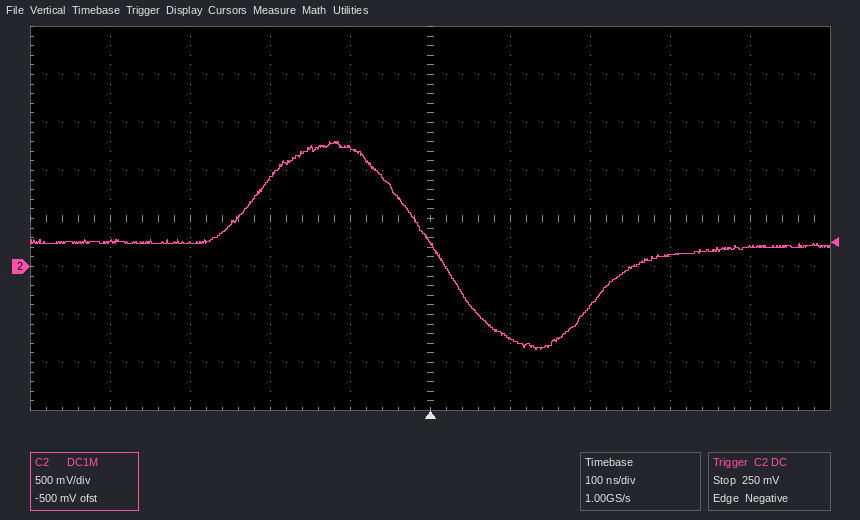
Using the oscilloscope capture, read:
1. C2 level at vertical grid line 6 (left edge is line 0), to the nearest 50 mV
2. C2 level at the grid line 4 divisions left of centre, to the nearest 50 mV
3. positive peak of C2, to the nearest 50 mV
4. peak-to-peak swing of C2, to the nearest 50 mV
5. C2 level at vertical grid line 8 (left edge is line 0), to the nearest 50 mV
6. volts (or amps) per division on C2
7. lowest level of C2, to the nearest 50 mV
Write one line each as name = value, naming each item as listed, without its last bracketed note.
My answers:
C2 level at vertical grid line 6 (left edge is line 0), to the nearest 50 mV = -750 mV
C2 level at the grid line 4 divisions left of centre, to the nearest 50 mV = 250 mV
positive peak of C2, to the nearest 50 mV = 1.30 V
peak-to-peak swing of C2, to the nearest 50 mV = 2.15 V
C2 level at vertical grid line 8 (left edge is line 0), to the nearest 50 mV = 100 mV
volts (or amps) per division on C2 = 500 mV
lowest level of C2, to the nearest 50 mV = -850 mV
